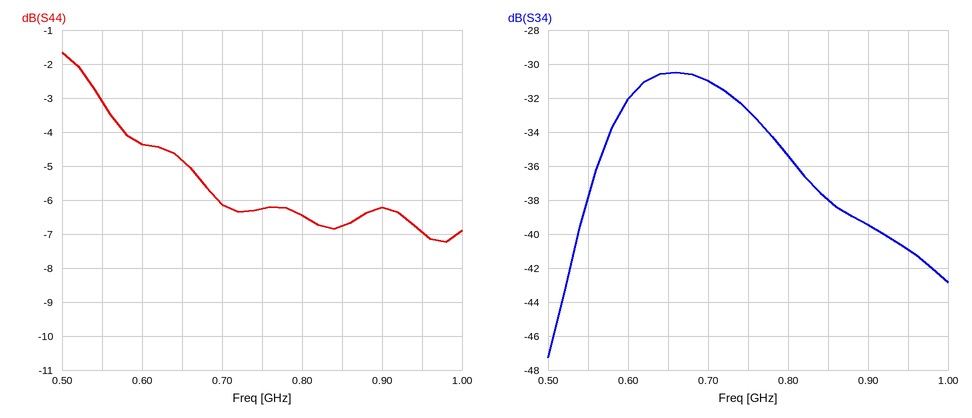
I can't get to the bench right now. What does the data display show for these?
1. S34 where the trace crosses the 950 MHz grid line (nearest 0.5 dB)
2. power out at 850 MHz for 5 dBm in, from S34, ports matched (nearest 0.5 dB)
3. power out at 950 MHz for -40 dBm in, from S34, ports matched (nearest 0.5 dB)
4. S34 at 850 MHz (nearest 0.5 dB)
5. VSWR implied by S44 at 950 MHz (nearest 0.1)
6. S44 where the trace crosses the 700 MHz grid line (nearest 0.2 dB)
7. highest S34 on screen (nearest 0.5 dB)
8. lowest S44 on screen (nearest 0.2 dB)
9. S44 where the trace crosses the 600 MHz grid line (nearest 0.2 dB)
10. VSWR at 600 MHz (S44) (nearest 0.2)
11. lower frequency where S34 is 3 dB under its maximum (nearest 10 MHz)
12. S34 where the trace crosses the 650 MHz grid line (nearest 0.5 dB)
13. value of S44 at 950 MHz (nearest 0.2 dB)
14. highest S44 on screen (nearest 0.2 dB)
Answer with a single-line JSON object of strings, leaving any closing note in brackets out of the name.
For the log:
{"S34 where the trace crosses the 950 MHz grid line": "-41.0 dB", "power out at 850 MHz for 5 dBm in, from S34, ports matched": "-33.0 dBm", "power out at 950 MHz for -40 dBm in, from S34, ports matched": "-81.0 dBm", "S34 at 850 MHz": "-38.0 dB", "VSWR implied by S44 at 950 MHz": "2.6", "S44 where the trace crosses the 700 MHz grid line": "-6.2 dB", "highest S34 on screen": "-30.5 dB", "lowest S44 on screen": "-7.2 dB", "S44 where the trace crosses the 600 MHz grid line": "-4.4 dB", "VSWR at 600 MHz (S44)": "4.0", "lower frequency where S34 is 3 dB under its maximum": "580 MHz", "S34 where the trace crosses the 650 MHz grid line": "-30.5 dB", "value of S44 at 950 MHz": "-7.0 dB", "highest S44 on screen": "-1.6 dB"}
